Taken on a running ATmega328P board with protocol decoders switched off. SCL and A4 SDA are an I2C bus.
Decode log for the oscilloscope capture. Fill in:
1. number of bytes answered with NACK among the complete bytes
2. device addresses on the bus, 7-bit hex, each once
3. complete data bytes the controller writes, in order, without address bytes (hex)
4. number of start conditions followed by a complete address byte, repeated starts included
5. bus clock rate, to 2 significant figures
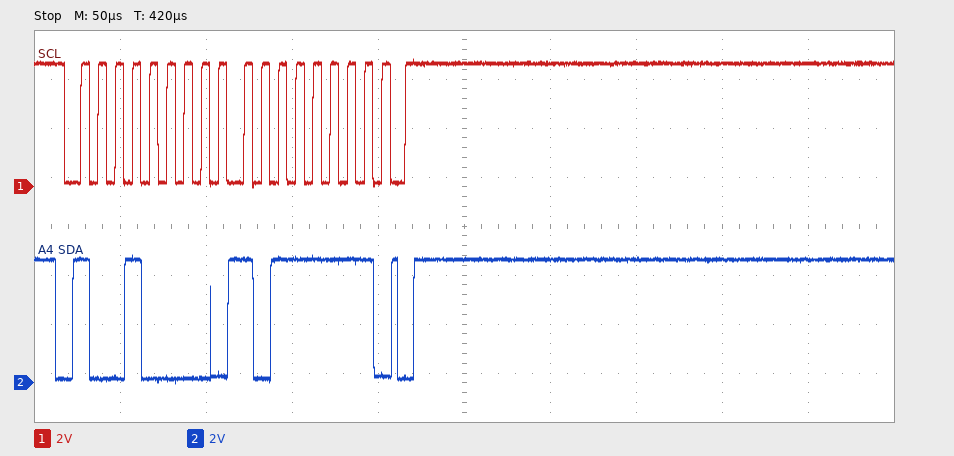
0
0x48
BF
1
100 kHz
